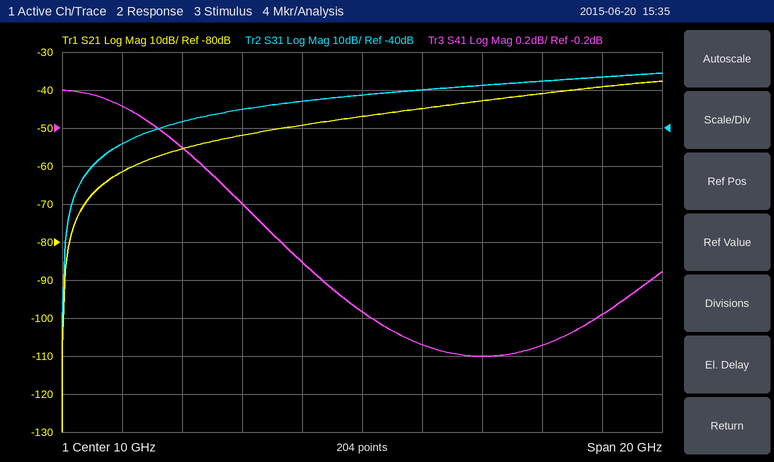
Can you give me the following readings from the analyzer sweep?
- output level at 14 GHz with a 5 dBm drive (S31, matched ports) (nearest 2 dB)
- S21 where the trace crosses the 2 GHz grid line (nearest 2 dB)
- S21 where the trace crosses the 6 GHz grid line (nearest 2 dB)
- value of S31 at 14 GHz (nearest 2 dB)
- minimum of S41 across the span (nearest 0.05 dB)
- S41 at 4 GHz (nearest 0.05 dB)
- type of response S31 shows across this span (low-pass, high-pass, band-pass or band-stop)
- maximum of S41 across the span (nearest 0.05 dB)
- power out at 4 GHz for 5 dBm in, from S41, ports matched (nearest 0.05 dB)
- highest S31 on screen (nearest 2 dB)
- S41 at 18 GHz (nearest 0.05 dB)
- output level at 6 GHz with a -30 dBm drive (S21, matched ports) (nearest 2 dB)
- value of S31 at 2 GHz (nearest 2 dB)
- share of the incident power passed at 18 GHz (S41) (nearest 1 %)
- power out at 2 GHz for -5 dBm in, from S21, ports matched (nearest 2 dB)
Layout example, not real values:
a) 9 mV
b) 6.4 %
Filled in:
a) -24 dBm
b) -62 dB
c) -52 dB
d) -28 dB
e) -1.40 dB
f) -0.30 dB
g) high-pass
h) 0.00 dB
i) 4.70 dBm
j) -26 dB
k) -1.20 dB
l) -82 dBm
m) -44 dB
n) 76 %
o) -66 dBm
